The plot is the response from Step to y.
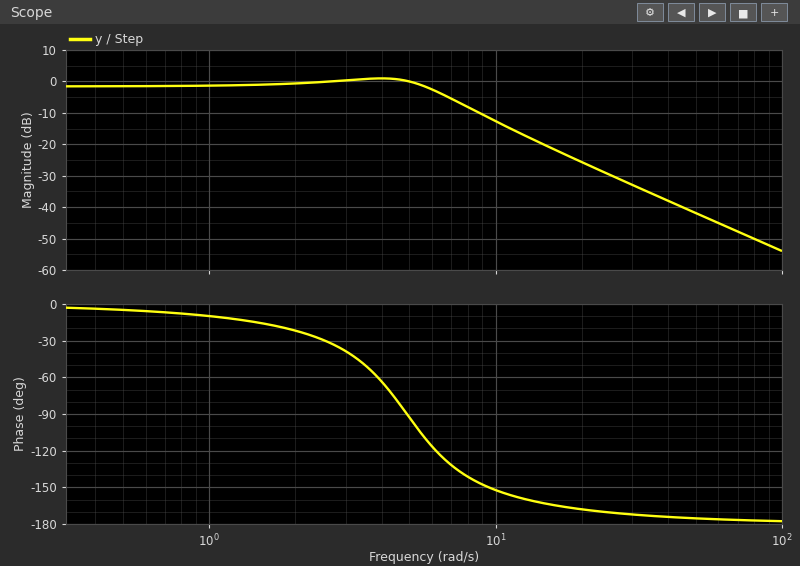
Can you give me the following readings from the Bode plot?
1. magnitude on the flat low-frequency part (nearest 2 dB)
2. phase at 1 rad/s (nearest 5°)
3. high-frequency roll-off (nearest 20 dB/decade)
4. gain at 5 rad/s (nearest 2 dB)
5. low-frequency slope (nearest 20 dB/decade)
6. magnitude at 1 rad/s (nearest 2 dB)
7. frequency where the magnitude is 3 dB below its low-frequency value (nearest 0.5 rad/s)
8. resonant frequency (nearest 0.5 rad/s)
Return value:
-2 dB
-10°
-40 dB/decade
0 dB
0 dB/decade
-2 dB
6.5 rad/s
4.0 rad/s
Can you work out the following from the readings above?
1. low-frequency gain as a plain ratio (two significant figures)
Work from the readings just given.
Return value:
0.79
